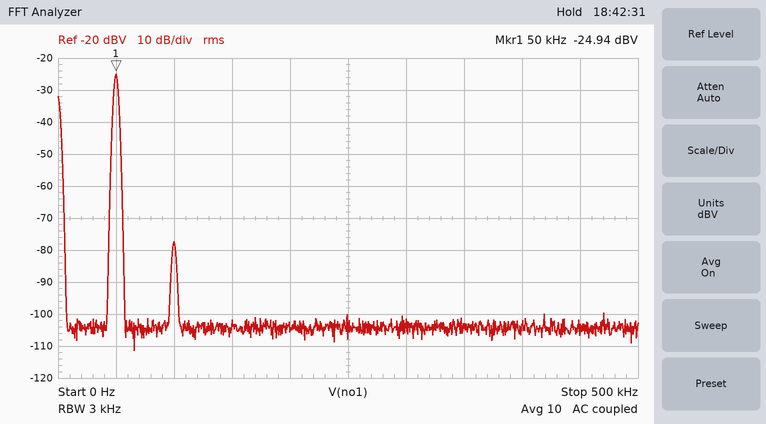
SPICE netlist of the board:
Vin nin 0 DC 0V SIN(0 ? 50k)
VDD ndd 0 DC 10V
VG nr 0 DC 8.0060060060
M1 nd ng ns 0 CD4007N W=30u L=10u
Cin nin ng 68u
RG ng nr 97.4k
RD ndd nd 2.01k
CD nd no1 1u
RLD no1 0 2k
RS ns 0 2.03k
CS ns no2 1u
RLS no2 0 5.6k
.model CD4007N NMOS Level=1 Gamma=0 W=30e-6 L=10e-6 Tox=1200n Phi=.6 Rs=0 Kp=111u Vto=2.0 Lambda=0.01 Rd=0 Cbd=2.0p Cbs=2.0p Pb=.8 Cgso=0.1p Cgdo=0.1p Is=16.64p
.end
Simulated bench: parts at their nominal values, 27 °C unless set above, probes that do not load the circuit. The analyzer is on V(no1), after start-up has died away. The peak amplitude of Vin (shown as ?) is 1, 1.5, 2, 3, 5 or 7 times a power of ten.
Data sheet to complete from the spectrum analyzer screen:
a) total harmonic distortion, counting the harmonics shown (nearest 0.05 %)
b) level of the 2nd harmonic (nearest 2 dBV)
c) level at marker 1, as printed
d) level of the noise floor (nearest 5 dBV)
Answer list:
0.25 %
-78 dBV
-24.94 dBV
-105 dBV
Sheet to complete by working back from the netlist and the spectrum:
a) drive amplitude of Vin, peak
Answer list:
200 mV
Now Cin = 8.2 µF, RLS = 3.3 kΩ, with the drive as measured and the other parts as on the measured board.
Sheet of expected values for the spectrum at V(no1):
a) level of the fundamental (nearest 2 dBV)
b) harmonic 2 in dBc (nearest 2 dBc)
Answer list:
-24 dBV
-50 dBc
